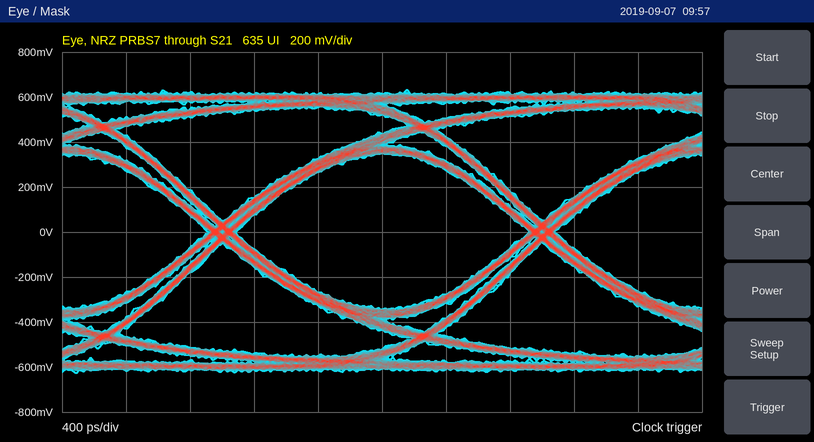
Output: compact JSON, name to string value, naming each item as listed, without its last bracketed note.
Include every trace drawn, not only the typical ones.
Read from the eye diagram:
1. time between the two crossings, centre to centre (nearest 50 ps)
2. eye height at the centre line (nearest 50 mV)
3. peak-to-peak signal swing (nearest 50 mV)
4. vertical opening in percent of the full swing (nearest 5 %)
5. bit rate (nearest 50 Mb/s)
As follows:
{"time between the two crossings, centre to centre": "2.00 ns", "eye height at the centre line": "700 mV", "peak-to-peak signal swing": "1.25 V", "vertical opening in percent of the full swing": "55 %", "bit rate": "500 Mb/s"}
